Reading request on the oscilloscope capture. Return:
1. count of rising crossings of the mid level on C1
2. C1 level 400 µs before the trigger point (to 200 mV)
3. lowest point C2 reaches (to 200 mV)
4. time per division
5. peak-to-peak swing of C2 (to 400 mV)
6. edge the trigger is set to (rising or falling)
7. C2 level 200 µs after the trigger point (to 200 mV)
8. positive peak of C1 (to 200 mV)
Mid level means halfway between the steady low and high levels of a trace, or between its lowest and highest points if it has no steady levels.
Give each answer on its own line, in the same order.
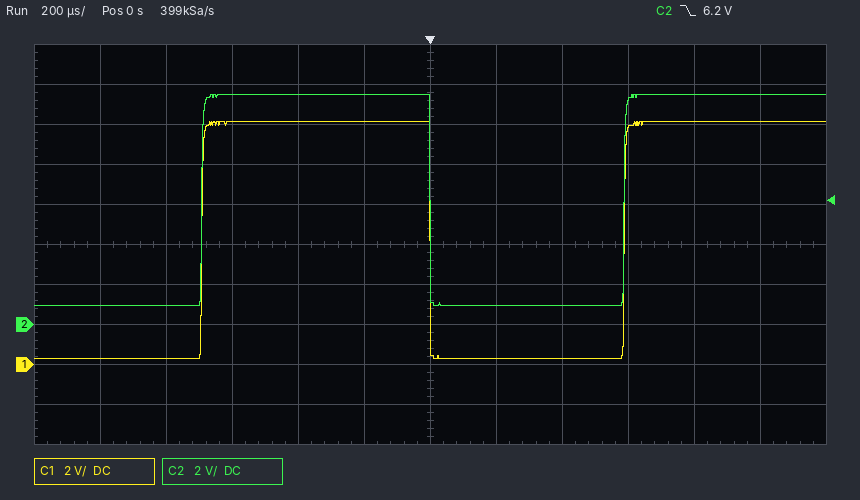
2
12.2 V
1.0 V
200 µs
10.4 V
falling
1.0 V
12.2 V
